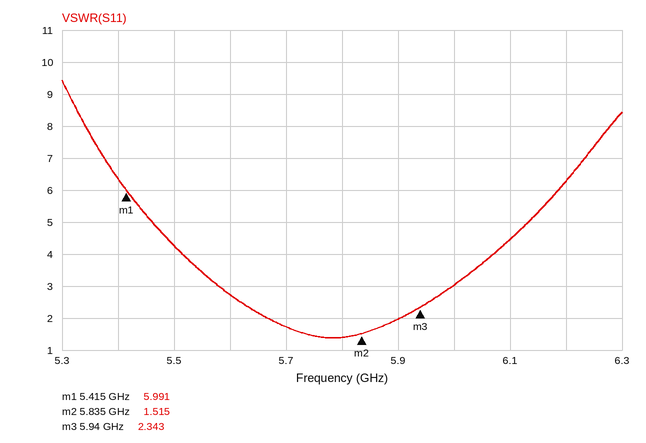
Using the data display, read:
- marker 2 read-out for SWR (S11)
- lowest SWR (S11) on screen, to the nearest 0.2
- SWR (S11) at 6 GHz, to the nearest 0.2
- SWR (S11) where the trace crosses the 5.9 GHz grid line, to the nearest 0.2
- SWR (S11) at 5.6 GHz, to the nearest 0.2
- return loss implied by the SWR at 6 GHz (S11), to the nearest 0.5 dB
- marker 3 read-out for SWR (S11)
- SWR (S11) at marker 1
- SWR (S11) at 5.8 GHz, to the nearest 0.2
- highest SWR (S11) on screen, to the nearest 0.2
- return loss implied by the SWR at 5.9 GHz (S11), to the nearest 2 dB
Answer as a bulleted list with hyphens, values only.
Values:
- 1.515
- 1.4
- 3.0
- 2.0
- 2.8
- 6.0 dB
- 2.343
- 5.991
- 1.4
- 9.4
- 10 dB
